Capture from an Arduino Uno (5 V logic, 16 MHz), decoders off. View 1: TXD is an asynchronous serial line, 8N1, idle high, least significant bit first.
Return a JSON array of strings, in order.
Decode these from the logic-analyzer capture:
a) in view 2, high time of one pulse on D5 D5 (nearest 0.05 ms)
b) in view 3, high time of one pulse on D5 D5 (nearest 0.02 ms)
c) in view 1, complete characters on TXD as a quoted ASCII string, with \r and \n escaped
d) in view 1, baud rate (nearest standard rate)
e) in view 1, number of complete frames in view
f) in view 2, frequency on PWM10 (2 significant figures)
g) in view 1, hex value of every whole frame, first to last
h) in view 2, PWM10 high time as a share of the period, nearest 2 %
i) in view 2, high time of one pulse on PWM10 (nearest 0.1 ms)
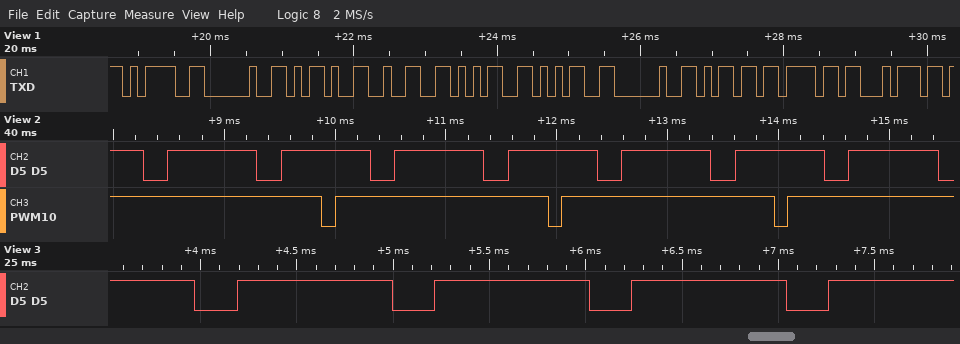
["0.80 ms", "0.80 ms", "\"= -255 mot\"", "9600 baud", "10", "490 Hz", "0x3D 0x20 0x2D 0x32 0x35 0x35 0x20 0x6D 0x6F 0x74", "94 %", "1.9 ms"]
